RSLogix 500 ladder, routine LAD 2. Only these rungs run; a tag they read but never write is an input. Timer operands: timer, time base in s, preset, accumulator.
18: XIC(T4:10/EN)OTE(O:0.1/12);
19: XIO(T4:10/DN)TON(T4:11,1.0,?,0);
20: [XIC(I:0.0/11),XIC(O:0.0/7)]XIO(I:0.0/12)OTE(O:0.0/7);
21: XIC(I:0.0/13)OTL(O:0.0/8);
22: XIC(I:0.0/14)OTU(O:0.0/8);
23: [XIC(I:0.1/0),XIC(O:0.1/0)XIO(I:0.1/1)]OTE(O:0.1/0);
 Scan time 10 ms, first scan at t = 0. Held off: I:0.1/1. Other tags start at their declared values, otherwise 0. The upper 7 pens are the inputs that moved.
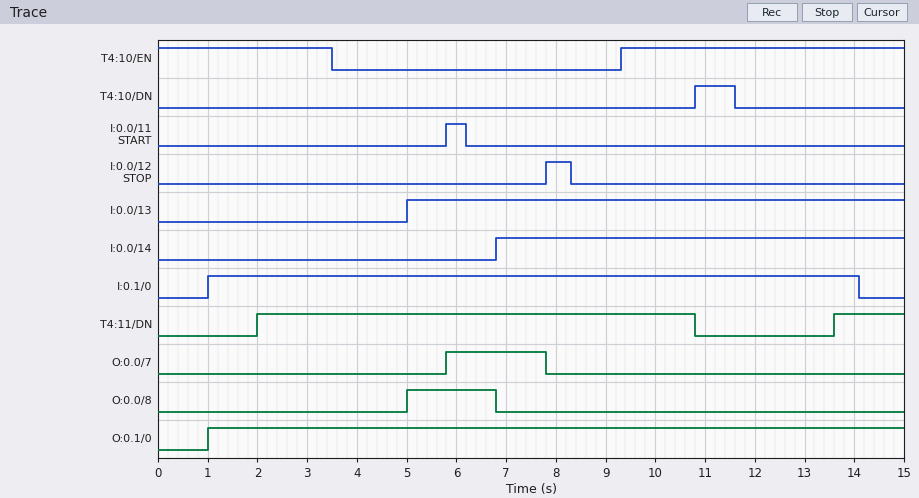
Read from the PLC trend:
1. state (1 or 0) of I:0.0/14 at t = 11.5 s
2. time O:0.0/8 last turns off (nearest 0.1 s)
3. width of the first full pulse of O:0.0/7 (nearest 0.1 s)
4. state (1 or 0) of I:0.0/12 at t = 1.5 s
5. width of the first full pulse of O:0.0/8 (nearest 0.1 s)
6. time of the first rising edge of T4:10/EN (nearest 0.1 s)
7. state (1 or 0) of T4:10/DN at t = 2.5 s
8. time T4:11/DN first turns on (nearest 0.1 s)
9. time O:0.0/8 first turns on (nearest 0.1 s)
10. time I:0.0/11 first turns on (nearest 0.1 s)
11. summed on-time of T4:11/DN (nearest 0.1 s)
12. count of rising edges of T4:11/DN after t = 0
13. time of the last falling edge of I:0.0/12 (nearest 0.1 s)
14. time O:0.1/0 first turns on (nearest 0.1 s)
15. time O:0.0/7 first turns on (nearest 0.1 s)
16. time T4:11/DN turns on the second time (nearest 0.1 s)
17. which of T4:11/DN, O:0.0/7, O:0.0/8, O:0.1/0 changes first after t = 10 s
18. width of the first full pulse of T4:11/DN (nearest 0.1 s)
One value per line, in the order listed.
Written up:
1
6.8 s
2.0 s
0
1.8 s
9.3 s
0
2.0 s
5.0 s
5.8 s
10.2 s
2
8.3 s
1.0 s
5.8 s
13.6 s
T4:11/DN
8.8 s
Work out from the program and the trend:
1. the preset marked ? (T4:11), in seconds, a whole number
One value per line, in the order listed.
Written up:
2 s
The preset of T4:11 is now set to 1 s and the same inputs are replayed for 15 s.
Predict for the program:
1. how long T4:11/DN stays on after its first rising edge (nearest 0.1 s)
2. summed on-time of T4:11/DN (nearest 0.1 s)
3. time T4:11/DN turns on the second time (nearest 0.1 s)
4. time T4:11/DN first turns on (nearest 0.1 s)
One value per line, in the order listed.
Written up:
9.8 s
12.2 s
12.6 s
1.0 s
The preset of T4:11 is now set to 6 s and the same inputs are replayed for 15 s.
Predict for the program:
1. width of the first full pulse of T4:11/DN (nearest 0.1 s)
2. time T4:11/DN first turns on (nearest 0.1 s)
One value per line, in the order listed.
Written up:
4.8 s
6.0 s
